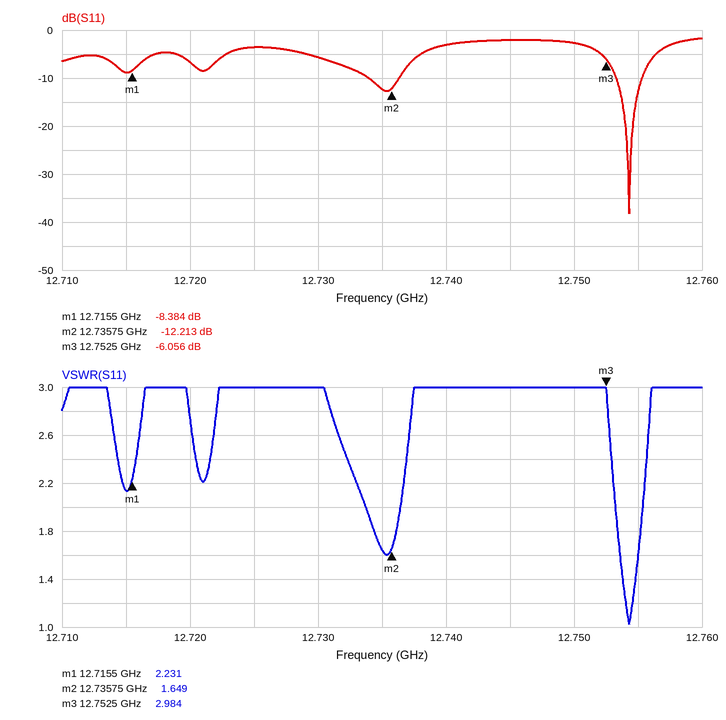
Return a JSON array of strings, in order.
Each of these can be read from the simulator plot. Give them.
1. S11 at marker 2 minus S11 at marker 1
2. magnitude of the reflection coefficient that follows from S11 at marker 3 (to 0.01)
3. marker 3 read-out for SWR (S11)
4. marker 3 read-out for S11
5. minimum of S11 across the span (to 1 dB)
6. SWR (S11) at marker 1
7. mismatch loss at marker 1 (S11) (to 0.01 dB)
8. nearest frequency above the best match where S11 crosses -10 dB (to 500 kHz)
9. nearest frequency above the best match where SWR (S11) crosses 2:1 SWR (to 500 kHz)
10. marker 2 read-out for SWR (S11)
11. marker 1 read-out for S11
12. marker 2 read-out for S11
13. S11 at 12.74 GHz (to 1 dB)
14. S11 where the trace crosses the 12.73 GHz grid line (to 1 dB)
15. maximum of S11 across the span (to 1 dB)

["-3.829 dB", "0.50", "2.984", "-6.056 dB", "-38 dB", "2.231", "0.68 dB", "12.7555 GHz", "12.7555 GHz", "1.649", "-8.384 dB", "-12.213 dB", "-3 dB", "-6 dB", "-2 dB"]
